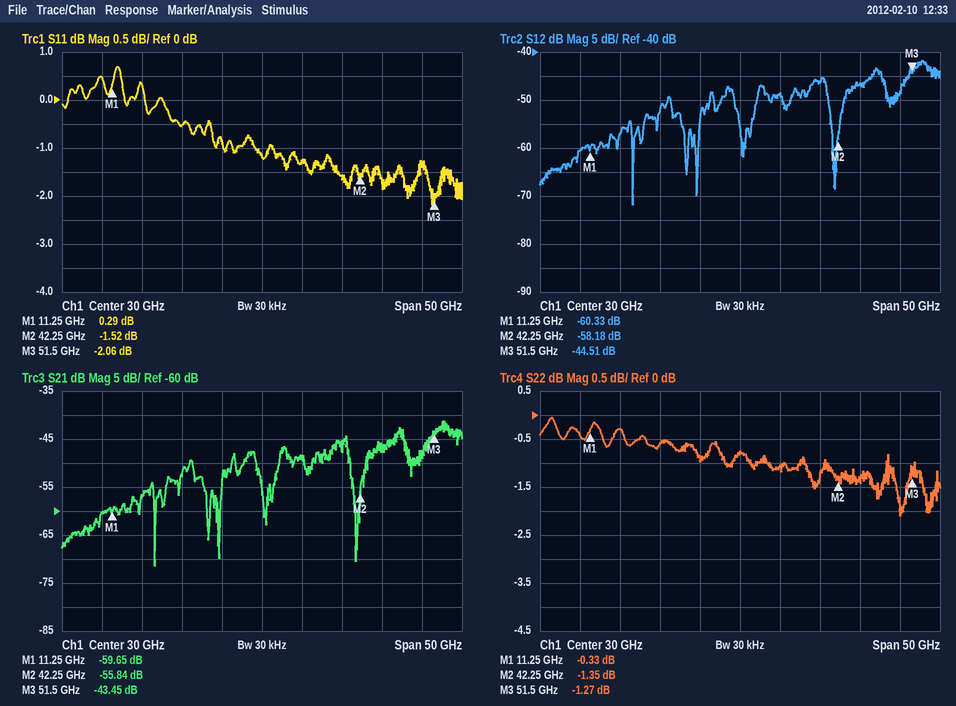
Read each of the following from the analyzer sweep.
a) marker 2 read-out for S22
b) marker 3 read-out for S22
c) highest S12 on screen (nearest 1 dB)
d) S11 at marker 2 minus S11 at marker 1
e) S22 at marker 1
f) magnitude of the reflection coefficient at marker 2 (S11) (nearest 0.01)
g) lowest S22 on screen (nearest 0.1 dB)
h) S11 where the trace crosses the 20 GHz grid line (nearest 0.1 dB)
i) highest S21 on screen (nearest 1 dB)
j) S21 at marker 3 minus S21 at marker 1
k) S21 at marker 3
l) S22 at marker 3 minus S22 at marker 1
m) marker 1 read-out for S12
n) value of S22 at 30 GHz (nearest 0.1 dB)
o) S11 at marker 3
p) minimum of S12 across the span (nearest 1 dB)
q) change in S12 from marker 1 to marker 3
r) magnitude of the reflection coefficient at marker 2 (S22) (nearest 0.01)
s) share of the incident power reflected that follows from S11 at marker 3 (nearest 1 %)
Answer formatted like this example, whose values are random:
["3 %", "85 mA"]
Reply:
["-1.35 dB", "-1.27 dB", "-42 dB", "-1.81 dB", "-0.33 dB", "0.84", "-2.1 dB", "-0.5 dB", "-41 dB", "16.20 dB", "-43.45 dB", "-0.94 dB", "-60.33 dB", "-0.8 dB", "-2.06 dB", "-72 dB", "15.82 dB", "0.86", "62 %"]
